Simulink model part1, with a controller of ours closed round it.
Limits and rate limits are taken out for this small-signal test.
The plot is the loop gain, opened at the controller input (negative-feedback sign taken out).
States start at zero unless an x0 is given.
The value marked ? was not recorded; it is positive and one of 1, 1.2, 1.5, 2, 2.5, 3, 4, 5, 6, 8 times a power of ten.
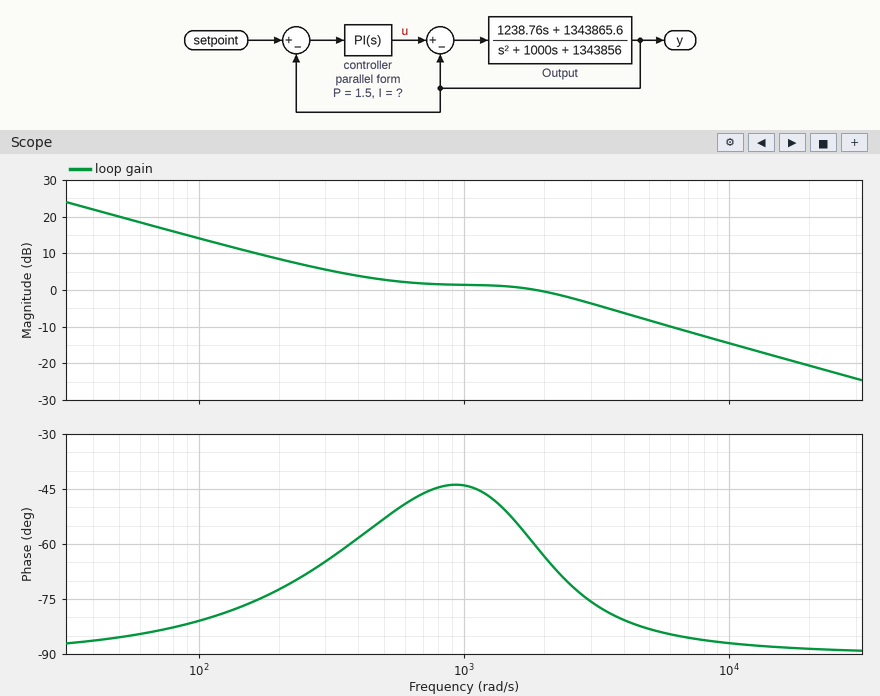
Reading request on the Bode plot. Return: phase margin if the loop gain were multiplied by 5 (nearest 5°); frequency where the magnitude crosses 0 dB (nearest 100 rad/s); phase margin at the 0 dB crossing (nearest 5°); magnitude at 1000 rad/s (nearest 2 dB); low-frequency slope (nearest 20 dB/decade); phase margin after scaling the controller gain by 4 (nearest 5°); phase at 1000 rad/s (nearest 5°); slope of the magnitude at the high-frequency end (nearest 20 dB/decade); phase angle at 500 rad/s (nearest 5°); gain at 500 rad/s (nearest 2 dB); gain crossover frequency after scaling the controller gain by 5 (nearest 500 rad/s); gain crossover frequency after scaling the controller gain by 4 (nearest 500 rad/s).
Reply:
95°
1900 rad/s
120°
2 dB
-20 dB/decade
95°
-45°
-20 dB/decade
-55°
2 dB
9500 rad/s
7500 rad/s
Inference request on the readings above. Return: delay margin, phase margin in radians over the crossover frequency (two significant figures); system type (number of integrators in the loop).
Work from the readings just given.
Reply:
0.0011 s
1
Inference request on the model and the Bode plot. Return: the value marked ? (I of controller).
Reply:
1000
